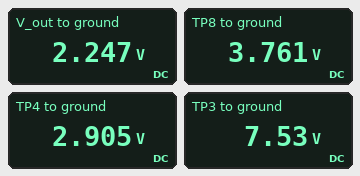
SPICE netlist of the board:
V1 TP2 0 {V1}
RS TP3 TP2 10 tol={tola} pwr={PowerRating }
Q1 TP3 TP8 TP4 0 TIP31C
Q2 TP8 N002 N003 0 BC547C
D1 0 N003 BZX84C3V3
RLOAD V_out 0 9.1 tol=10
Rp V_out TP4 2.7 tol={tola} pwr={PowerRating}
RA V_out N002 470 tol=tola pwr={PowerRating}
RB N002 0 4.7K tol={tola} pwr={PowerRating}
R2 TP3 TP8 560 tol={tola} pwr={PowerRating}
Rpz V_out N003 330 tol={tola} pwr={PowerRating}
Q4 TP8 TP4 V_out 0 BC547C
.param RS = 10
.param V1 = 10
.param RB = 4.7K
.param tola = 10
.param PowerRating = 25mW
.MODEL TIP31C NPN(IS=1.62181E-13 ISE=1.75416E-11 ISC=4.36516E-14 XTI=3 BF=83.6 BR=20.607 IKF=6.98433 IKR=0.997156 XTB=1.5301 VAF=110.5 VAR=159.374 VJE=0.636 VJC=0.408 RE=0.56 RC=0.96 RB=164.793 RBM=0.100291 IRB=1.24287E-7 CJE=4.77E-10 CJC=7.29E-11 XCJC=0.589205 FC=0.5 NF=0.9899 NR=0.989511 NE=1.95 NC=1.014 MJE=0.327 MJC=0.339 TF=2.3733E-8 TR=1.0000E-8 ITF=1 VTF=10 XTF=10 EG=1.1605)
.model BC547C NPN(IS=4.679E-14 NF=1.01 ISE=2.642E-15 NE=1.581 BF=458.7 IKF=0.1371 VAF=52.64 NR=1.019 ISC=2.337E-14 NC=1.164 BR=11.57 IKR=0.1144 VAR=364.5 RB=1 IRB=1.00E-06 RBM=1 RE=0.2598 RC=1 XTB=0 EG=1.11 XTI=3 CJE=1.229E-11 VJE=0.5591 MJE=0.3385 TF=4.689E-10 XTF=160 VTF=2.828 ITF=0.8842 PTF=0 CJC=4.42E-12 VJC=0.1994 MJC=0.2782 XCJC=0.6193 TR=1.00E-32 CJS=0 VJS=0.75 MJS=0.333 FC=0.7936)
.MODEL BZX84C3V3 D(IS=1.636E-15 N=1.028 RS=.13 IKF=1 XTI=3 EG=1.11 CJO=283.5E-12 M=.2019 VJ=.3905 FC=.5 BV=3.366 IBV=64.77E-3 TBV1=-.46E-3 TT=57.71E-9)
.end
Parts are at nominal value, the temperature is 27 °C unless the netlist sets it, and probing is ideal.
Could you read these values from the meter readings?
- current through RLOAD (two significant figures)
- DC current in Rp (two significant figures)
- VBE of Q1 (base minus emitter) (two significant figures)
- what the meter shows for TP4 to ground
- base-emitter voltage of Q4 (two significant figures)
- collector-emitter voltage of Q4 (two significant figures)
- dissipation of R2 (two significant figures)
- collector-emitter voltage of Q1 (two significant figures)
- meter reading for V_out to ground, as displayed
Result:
250 mA
240 mA
860 mV
2.905 V
660 mV
1.5 V
25 mW
4.6 V
2.247 V
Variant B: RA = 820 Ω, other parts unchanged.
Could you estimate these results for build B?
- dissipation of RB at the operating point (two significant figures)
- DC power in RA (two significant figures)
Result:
780 µW
140 µW
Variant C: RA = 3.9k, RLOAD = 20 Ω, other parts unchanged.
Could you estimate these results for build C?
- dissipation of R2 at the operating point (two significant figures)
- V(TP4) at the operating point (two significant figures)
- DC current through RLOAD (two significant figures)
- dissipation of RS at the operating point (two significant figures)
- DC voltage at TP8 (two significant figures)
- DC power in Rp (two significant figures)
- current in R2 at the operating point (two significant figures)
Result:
6.2 mW
5.0 V
220 mA
510 mW
5.9 V
140 mW
3.3 mA
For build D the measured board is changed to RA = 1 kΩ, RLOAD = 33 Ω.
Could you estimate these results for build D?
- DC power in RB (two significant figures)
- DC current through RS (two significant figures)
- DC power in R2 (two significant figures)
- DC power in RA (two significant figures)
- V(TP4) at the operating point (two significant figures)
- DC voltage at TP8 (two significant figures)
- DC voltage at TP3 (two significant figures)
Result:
3.3 mW
150 mA
11 mW
720 µW
5.2 V
6.0 V
8.5 V
